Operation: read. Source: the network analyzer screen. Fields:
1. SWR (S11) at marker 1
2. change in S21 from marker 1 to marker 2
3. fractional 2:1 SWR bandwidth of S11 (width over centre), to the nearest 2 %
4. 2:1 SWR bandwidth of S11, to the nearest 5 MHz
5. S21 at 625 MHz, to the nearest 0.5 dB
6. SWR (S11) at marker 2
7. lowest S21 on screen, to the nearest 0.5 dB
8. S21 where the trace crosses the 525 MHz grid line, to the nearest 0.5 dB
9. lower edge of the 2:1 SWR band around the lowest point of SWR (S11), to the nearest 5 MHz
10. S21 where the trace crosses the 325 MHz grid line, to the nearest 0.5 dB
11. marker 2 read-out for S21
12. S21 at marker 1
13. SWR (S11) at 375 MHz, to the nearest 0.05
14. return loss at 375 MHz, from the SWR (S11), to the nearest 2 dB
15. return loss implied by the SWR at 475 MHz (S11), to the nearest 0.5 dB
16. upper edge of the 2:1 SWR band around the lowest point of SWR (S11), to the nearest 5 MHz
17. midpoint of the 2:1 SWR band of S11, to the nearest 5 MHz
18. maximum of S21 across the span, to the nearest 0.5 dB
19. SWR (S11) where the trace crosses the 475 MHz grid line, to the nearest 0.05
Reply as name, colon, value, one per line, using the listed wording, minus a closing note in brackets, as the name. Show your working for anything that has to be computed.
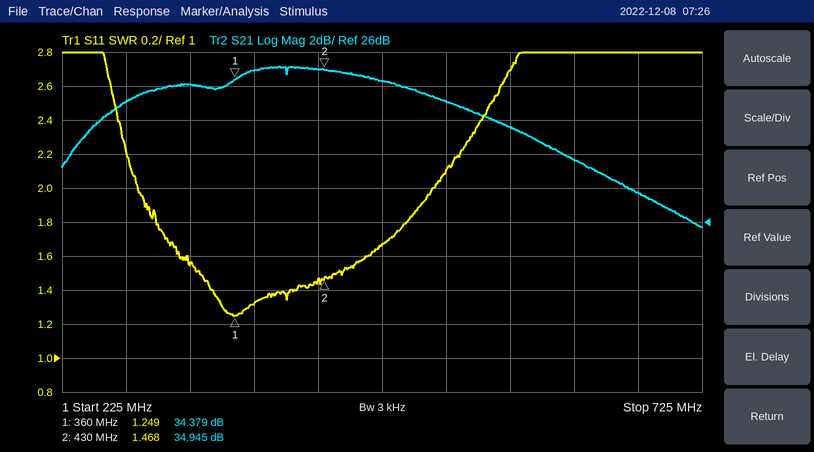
SWR (S11) at marker 1: 1.249
change in S21 from marker 1 to marker 2: 34.945 − (34.379) = 0.566 dB
fractional 2:1 SWR bandwidth of S11 (width over centre), to the nearest 2 %: 230 MHz / 400 MHz ≈ 58 %
2:1 SWR bandwidth of S11, to the nearest 5 MHz: 515 MHz − 285 MHz = 230 MHz
S21 at 625 MHz, to the nearest 0.5 dB: 29.5 dB
SWR (S11) at marker 2: 1.468
lowest S21 on screen, to the nearest 0.5 dB: 25.5 dB
S21 where the trace crosses the 525 MHz grid line, to the nearest 0.5 dB: 33.0 dB
lower edge of the 2:1 SWR band around the lowest point of SWR (S11), to the nearest 5 MHz: 285 MHz
S21 where the trace crosses the 325 MHz grid line, to the nearest 0.5 dB: 34.0 dB
marker 2 read-out for S21: 34.945 dB
S21 at marker 1: 34.379 dB
SWR (S11) at 375 MHz, to the nearest 0.05: 1.30
return loss at 375 MHz, from the SWR (S11), to the nearest 2 dB: −20 log10((1.3 − 1)/(1.3 + 1)) ≈ 18 dB
return loss implied by the SWR at 475 MHz (S11), to the nearest 0.5 dB: −20 log10((1.65 − 1)/(1.65 + 1)) ≈ 12.2 dB, so 12.0 dB to the nearest 0.5 dB
upper edge of the 2:1 SWR band around the lowest point of SWR (S11), to the nearest 5 MHz: 515 MHz
midpoint of the 2:1 SWR band of S11, to the nearest 5 MHz: 400 MHz
maximum of S21 across the span, to the nearest 0.5 dB: 35.0 dB
SWR (S11) where the trace crosses the 475 MHz grid line, to the nearest 0.05: 1.65
